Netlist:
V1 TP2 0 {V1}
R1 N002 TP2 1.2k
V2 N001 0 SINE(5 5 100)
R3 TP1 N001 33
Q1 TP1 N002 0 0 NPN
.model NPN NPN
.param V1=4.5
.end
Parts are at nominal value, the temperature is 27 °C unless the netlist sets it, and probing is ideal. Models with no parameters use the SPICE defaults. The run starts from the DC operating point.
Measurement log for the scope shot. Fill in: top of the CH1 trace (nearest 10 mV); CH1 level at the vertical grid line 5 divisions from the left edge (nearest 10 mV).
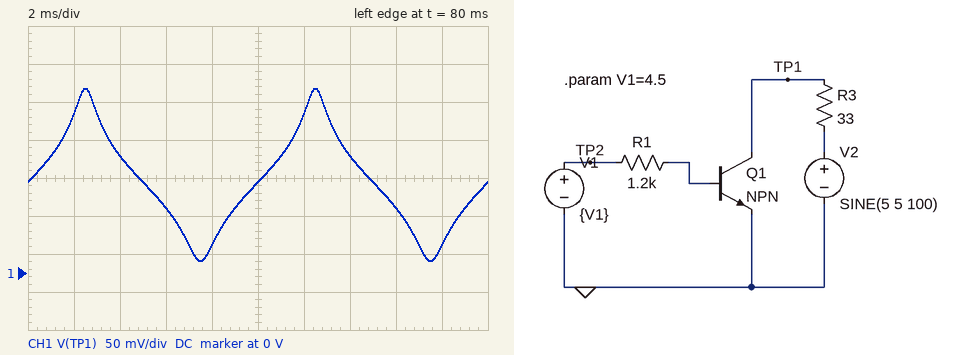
240 mV
120 mV
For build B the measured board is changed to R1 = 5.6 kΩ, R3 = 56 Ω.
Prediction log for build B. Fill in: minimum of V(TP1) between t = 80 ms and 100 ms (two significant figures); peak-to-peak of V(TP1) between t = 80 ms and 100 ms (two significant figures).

13 mV
6.4 V
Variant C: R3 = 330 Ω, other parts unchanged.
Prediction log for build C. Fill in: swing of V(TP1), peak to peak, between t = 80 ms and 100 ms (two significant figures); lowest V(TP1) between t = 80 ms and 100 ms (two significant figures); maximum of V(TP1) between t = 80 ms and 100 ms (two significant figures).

49 mV
18 mV
67 mV
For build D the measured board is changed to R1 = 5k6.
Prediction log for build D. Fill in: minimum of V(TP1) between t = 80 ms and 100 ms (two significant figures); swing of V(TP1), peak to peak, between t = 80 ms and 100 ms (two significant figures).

11 mV
7.9 V
